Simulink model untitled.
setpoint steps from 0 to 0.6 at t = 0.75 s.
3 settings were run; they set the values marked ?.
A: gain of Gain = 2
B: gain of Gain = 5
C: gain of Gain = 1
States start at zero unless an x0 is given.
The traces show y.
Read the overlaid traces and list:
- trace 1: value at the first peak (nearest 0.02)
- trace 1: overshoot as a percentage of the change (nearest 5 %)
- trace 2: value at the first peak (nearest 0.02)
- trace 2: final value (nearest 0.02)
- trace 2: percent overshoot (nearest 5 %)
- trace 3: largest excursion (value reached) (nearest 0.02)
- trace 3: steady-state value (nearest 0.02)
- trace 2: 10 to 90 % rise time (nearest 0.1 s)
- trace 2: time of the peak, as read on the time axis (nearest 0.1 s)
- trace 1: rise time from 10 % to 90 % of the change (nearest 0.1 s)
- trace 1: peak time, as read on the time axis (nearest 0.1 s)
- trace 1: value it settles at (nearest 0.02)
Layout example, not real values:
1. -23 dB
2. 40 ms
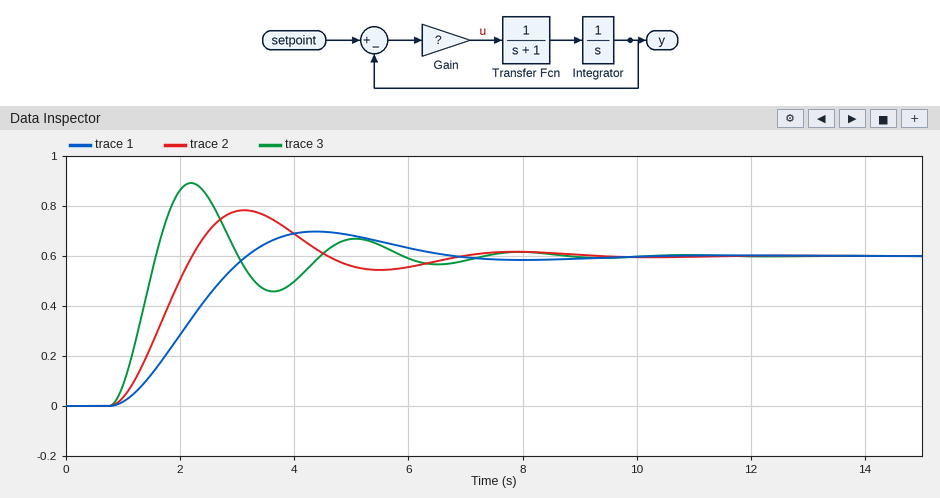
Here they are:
1. 0.70
2. 15 %
3. 0.78
4. 0.60
5. 30 %
6. 0.90
7. 0.60
8. 1.0 s
9. 3.1 s
10. 1.6 s
11. 4.4 s
12. 0.60
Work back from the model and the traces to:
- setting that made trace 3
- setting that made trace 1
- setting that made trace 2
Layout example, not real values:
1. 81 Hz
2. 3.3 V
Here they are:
1. B
2. C
3. A
